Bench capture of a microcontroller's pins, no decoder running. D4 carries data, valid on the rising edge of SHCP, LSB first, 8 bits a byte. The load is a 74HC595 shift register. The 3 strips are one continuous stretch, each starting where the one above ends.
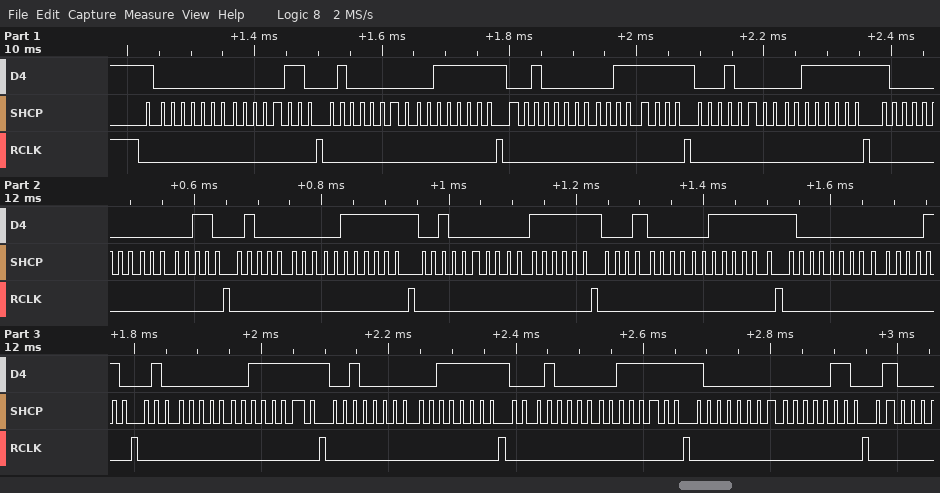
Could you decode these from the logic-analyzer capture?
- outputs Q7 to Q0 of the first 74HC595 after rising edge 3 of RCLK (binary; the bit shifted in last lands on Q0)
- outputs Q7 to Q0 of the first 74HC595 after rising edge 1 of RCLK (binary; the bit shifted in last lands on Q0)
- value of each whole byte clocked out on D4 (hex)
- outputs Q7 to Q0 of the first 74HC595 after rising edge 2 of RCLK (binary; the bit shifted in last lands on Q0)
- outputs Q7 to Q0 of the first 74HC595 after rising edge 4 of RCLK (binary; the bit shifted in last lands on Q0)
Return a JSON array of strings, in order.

["00111111", "00000110", "0x01 0x60 0x02 0xFC 0x04 0xFC 0x08 0xFC 0x01 0x60 0x02 0xFC 0x04 0xFC 0x08 0xFC 0x01 0x60 0x02 0xFC 0x04 0xFC 0x08 0xFC 0x01 0x60", "00111111", "00111111"]
